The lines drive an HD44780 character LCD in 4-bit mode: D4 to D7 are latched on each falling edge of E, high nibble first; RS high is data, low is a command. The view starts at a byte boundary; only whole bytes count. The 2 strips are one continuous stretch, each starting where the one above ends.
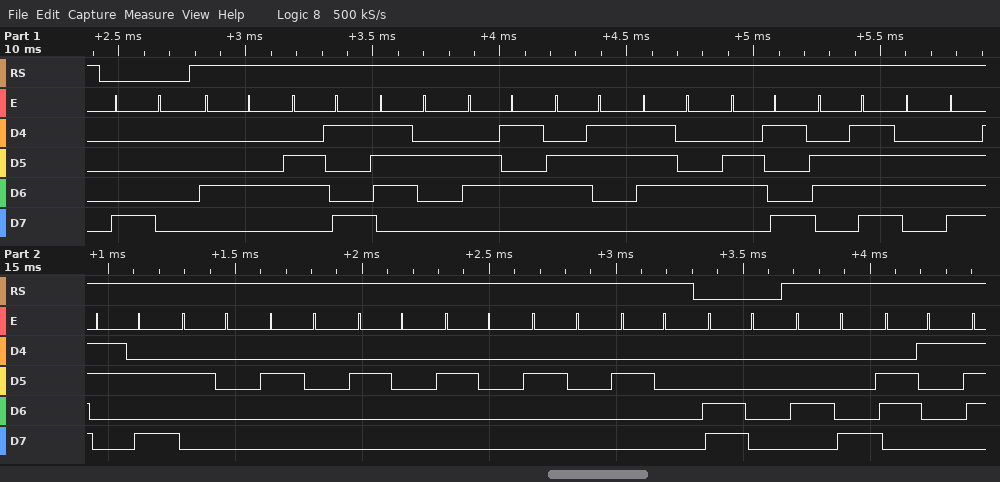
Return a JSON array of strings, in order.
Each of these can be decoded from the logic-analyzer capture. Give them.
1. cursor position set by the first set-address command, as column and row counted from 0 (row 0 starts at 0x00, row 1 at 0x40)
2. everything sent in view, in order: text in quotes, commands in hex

["column 0, row 0", "0x80 \"Direction:      \" 0xC0 \"Ha\""]
